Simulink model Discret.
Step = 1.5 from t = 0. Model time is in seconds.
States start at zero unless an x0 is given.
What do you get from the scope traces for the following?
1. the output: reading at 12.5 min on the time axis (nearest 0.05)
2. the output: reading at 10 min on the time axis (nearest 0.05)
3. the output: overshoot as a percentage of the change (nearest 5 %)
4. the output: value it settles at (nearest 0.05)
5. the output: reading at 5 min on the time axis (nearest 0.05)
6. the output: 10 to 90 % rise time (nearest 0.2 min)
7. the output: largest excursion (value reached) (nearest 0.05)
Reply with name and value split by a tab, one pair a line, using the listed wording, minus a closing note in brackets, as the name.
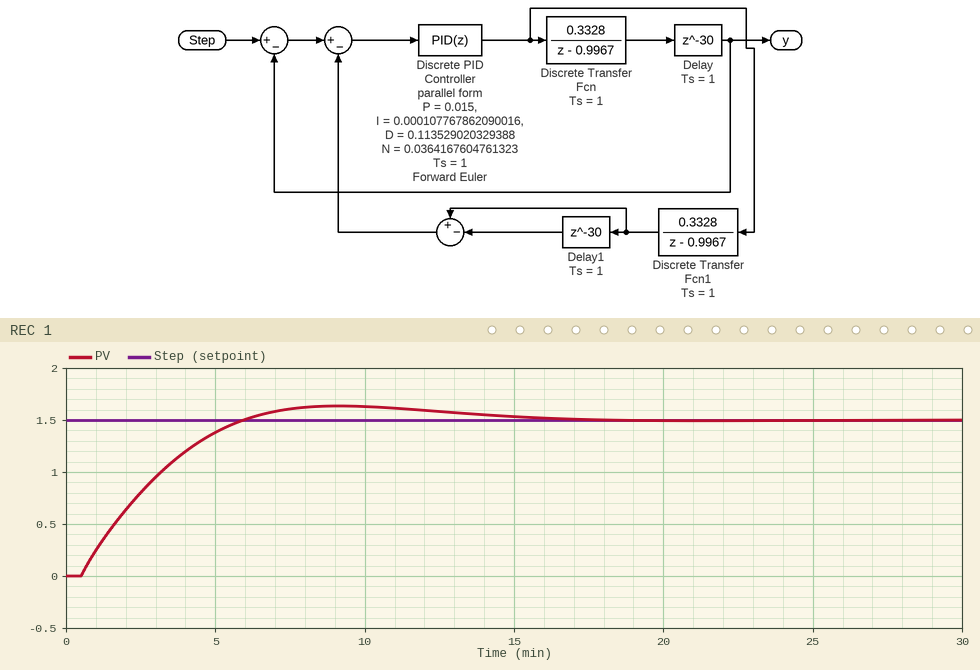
the output: reading at 12.5 min on the time axis	1.60
the output: reading at 10 min on the time axis	1.65
the output: overshoot as a percentage of the change	10 %
the output: value it settles at	1.50
the output: reading at 5 min on the time axis	1.40
the output: 10 to 90 % rise time	4.0 min
the output: largest excursion (value reached)	1.65
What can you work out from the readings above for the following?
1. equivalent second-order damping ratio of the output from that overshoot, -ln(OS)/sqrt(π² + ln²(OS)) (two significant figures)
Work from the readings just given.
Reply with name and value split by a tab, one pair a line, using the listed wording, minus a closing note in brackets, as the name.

equivalent second-order damping ratio of the output from that overshoot, -ln(OS)/sqrt(π² + ln²(OS))	0.59
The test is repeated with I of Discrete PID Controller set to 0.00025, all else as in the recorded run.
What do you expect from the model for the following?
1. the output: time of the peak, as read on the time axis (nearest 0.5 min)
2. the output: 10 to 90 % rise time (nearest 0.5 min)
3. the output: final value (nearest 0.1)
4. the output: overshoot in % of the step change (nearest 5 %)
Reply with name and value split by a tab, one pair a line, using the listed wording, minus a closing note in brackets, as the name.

the output: time of the peak, as read on the time axis	6.0 min
the output: 10 to 90 % rise time	2.5 min
the output: final value	1.5
the output: overshoot in % of the step change	25 %
